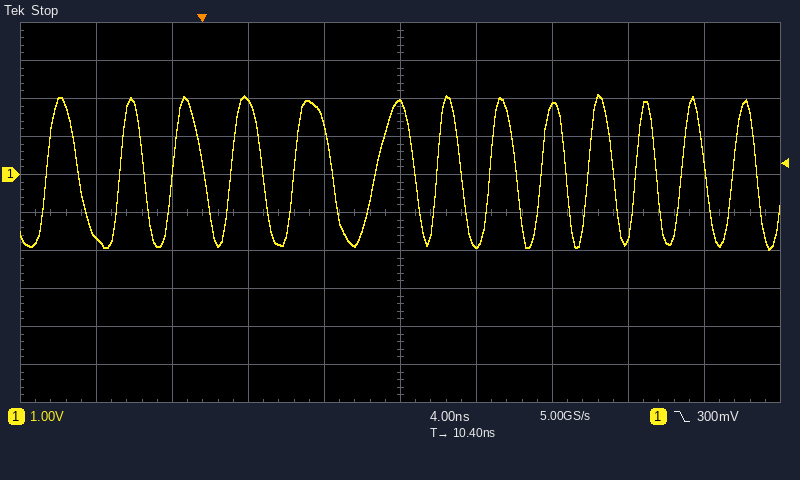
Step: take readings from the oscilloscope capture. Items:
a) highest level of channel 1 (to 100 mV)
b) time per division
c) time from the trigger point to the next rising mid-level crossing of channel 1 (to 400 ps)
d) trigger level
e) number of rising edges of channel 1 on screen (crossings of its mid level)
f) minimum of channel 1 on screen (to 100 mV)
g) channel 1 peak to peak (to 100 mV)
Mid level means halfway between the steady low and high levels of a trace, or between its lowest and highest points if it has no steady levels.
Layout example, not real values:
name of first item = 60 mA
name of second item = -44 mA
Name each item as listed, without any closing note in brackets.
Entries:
highest level of channel 1 = 2.1 V
time per division = 4 ns
time from the trigger point to the next rising mid-level crossing of channel 1 = 1.6 ns
trigger level = 300 mV
number of rising edges of channel 1 on screen = 13
minimum of channel 1 on screen = -2.0 V
channel 1 peak to peak = 4.1 V
